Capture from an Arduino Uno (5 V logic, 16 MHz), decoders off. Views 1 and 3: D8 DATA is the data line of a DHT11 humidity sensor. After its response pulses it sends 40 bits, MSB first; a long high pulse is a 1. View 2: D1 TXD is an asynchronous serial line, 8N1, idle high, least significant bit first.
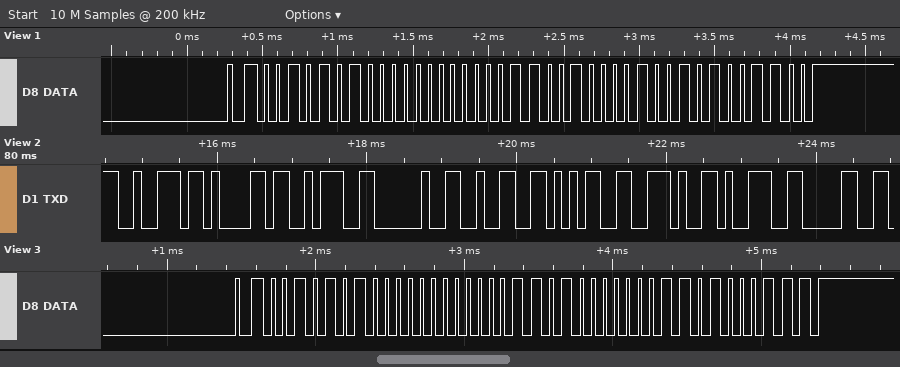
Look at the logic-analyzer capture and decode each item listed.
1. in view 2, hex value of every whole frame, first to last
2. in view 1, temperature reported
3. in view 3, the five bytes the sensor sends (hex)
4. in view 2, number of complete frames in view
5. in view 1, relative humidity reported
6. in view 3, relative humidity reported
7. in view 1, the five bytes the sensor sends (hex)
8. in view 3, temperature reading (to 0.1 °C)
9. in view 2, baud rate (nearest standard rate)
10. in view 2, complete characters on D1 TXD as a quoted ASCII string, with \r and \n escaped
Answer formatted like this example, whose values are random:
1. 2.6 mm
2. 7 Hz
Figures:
1. 72 61 3A 20 32 35 2E 39 30
2. 25.9 °C
3. 2A 00 1A 03 47
4. 9
5. 42 %
6. 42 %
7. 2A 00 19 09 4C
8. 26.3 °C
9. 9600 baud
10. "ra: 25.90"
